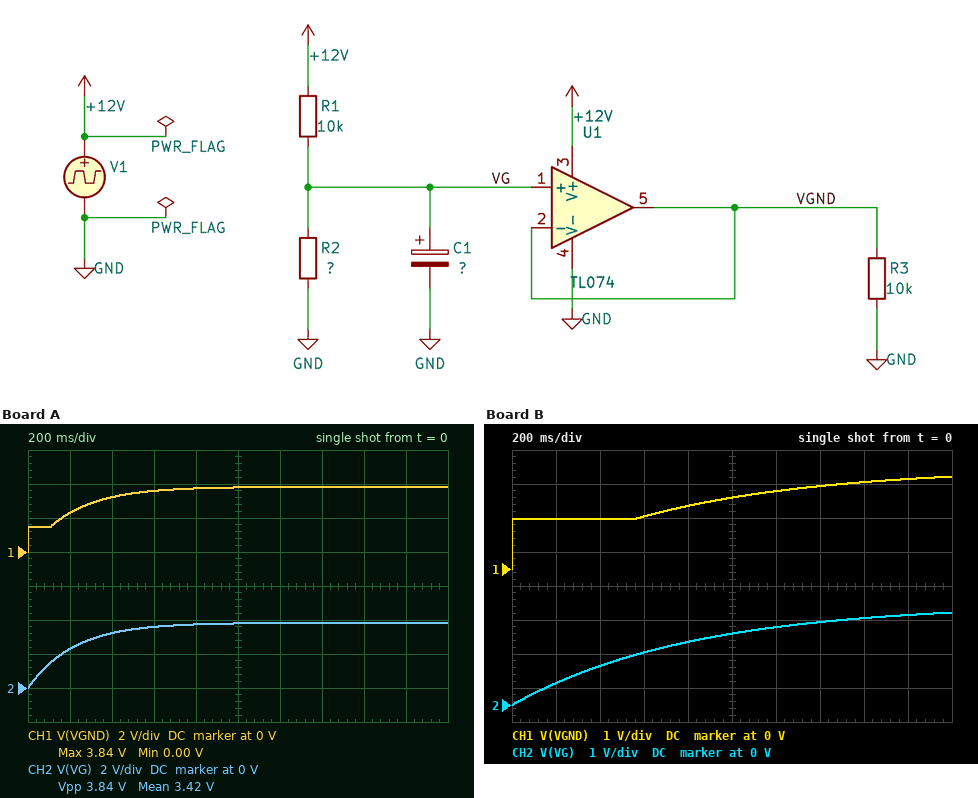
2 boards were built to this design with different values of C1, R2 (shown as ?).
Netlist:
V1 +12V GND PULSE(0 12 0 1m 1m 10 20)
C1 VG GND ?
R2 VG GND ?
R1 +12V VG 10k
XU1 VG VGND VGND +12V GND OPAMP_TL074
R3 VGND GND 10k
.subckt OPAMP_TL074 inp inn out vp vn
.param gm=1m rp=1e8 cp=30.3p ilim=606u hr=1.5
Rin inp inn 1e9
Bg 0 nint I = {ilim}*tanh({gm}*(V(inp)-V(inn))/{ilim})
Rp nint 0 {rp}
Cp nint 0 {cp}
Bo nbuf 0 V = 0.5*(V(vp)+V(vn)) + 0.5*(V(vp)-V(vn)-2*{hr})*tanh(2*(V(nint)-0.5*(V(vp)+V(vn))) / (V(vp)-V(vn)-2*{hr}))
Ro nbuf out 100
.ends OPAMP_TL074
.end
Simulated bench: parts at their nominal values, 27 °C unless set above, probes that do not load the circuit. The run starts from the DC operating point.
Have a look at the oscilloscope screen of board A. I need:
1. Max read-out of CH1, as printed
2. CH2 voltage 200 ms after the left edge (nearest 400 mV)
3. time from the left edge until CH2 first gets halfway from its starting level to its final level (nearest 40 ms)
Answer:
3.84 V
2.4 V
160 ms
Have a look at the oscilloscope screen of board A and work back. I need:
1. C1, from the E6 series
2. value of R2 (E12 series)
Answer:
68 µF
4.7 kΩ
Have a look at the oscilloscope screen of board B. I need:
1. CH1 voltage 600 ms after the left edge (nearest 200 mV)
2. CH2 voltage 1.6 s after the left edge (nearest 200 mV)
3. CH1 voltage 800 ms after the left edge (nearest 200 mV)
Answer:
1.6 V
2.6 V
1.8 V
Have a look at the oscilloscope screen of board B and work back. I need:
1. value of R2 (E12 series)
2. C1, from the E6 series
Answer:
3.3 kΩ
330 µF
